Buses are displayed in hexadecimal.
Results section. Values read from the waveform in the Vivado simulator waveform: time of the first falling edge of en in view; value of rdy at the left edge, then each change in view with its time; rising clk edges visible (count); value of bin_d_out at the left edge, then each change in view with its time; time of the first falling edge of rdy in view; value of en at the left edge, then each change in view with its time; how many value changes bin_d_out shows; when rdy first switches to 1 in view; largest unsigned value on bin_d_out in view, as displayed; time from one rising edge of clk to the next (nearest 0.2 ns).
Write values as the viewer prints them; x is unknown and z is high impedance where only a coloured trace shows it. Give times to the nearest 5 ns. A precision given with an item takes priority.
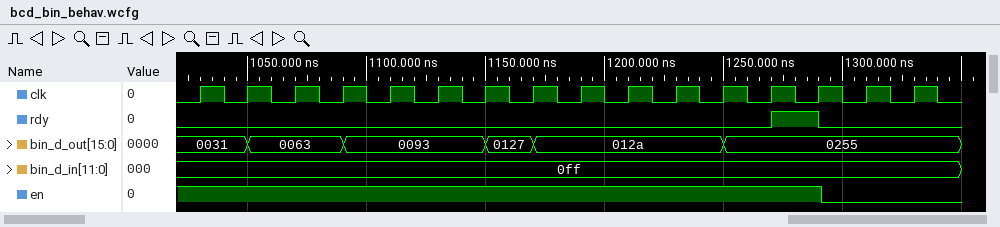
1290 ns
0, 1 at 1270 ns, 0 at 1290 ns
16
0031, 0063 at 1050 ns, 0093 at 1090 ns, 0127 at 1150 ns, 012a at 1170 ns, 0255 at 1250 ns
1290 ns
1, 0 at 1290 ns
5
1270 ns
0255
20 ns
